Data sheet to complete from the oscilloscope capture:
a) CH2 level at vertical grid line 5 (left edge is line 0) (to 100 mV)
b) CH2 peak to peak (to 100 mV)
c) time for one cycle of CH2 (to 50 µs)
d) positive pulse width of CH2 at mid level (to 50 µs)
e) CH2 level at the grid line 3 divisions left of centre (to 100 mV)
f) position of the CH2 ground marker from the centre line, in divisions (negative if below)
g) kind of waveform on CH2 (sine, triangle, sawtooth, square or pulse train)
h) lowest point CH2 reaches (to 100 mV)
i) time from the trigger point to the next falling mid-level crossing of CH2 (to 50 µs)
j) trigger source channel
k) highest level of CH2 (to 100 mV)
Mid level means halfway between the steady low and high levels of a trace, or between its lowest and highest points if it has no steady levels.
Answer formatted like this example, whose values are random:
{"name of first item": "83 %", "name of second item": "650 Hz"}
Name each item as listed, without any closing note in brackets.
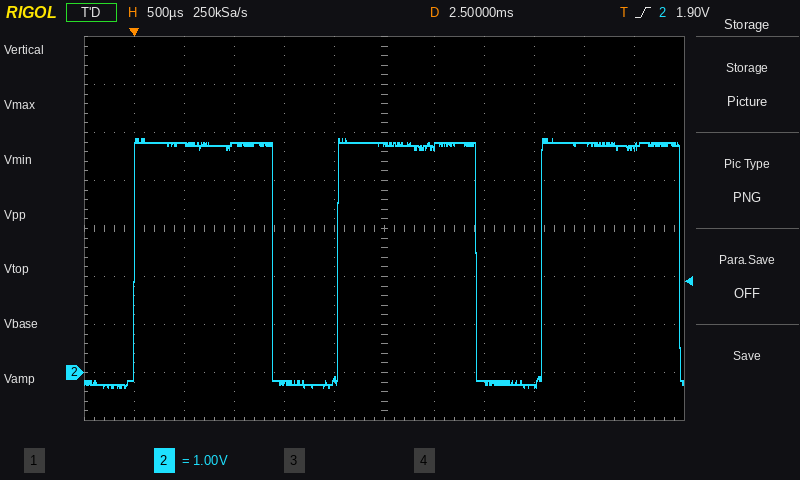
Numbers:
{"CH2 level at vertical grid line 5 (left edge is line 0)": "-200 mV", "CH2 peak to peak": "5.2 V", "time for one cycle of CH2": "2.05 ms", "positive pulse width of CH2 at mid level": "1.40 ms", "CH2 level at the grid line 3 divisions left of centre": "4.8 V", "position of the CH2 ground marker from the centre line, in divisions": "-3.0 div", "kind of waveform on CH2": "pulse train", "lowest point CH2 reaches": "-300 mV", "time from the trigger point to the next falling mid-level crossing of CH2": "1.40 ms", "trigger source channel": "CH2", "highest level of CH2": "4.9 V"}
